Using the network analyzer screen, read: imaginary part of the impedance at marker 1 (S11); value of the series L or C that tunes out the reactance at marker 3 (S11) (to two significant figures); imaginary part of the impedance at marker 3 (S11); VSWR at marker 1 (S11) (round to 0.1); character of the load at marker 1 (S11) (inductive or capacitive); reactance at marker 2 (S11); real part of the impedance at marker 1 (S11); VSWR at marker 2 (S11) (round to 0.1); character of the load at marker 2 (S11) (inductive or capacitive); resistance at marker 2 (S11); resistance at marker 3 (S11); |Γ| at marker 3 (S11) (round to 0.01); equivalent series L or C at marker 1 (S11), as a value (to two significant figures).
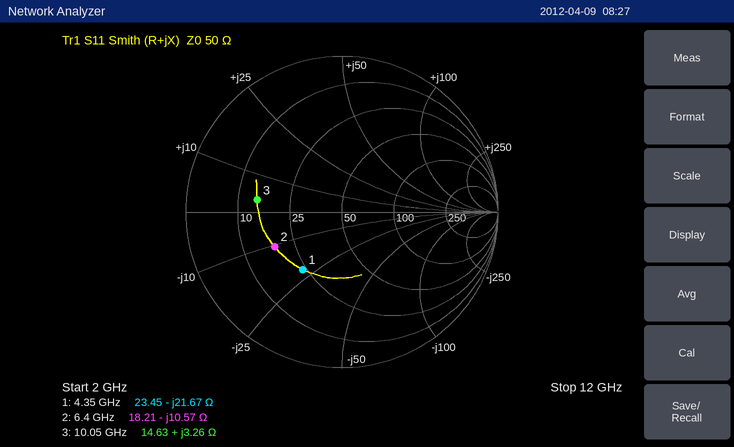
-21.67 Ω
4.9 pF
+3.26 Ω
2.6
capacitive
-10.57 Ω
23.45 Ω
2.9
capacitive
18.21 Ω
14.63 Ω
0.55
1.7 pF
